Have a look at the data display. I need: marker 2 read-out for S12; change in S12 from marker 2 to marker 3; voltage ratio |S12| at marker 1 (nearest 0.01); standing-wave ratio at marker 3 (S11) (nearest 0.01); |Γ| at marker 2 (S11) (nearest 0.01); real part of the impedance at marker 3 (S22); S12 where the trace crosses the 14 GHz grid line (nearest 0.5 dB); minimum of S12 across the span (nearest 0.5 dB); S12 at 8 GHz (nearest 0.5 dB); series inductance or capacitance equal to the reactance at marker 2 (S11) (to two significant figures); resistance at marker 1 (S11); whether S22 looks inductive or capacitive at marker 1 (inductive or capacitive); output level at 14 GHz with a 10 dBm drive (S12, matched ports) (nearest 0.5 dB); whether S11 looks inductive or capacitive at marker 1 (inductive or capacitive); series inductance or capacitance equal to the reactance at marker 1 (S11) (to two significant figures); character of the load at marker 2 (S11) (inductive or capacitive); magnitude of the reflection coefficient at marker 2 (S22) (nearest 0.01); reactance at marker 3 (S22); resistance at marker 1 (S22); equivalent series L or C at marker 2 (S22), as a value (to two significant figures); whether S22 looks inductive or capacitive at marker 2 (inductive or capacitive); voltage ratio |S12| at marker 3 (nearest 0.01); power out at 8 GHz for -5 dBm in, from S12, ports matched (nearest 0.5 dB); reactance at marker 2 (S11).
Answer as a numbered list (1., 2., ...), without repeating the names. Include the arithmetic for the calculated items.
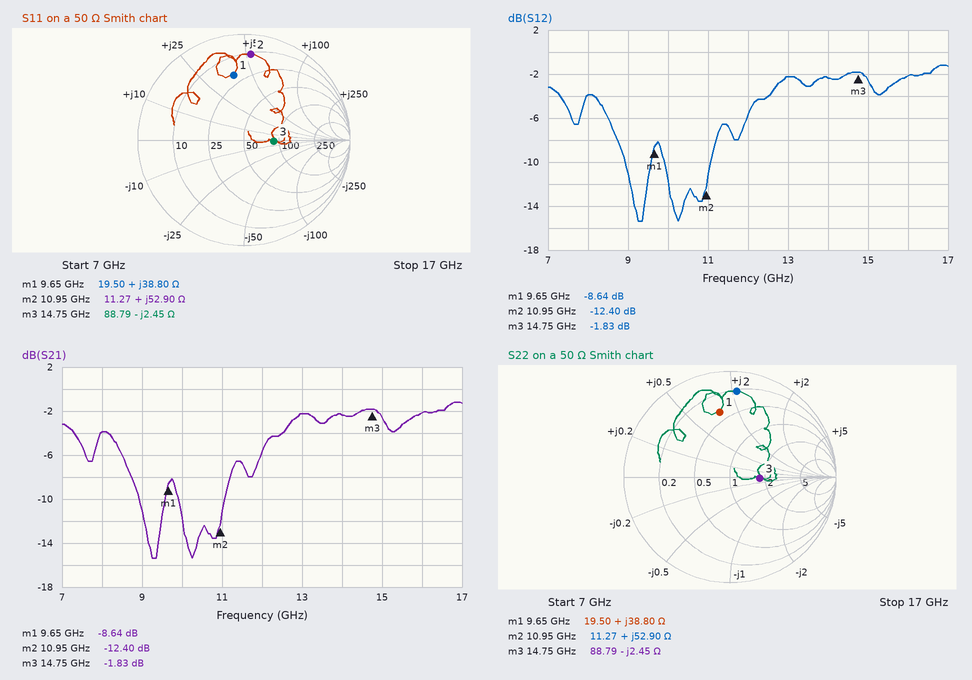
1. -12.40 dB
2. -1.83 − (-12.4) = 10.57 dB
3. 10^(-8.64/20) ≈ 0.37
4. 1.78
5. 0.81
6. 88.79 Ω
7. -2.5 dB
8. -15.5 dB
9. -4.0 dB
10. L = 52.9 Ω/(2π × 10.95 GHz) ≈ 769 pH, so 770 pH to two significant figures
11. 19.50 Ω
12. inductive
13. 10 dBm + (-2.5 dB) = 7.5 dBm
14. inductive
15. L = 38.8 Ω/(2π × 9.65 GHz) ≈ 640 pH
16. inductive
17. 0.81
18. -2.45 Ω
19. 19.50 Ω
20. L = 52.9 Ω/(2π × 10.95 GHz) ≈ 769 pH, so 770 pH to two significant figures
21. inductive
22. 10^(-1.83/20) ≈ 0.81
23. -5 dBm + (-4.0 dB) = -9.0 dBm
24. +52.90 Ω
